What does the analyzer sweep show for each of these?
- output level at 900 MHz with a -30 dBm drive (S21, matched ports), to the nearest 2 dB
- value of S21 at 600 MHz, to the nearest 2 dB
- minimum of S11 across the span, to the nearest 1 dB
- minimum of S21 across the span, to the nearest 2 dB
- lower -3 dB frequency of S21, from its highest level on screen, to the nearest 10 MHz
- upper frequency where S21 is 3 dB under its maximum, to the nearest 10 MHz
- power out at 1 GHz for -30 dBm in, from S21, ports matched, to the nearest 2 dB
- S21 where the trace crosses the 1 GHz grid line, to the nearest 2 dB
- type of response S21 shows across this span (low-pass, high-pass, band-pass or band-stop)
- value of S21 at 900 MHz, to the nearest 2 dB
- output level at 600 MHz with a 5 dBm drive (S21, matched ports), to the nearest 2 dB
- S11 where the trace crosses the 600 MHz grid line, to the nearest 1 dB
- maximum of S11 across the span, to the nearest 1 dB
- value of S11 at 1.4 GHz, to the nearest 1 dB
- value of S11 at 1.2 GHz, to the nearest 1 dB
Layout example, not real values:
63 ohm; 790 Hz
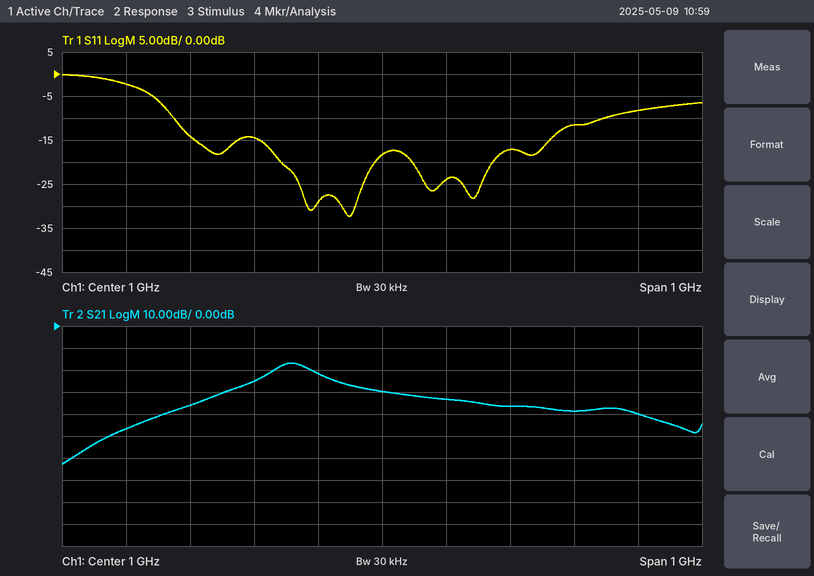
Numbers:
-52 dBm; -46 dB; -32 dB; -62 dB; 830 MHz; 890 MHz; -60 dBm; -30 dB; band-pass; -22 dB; -42 dBm; -2 dB; 0 dB; -8 dB; -17 dB
